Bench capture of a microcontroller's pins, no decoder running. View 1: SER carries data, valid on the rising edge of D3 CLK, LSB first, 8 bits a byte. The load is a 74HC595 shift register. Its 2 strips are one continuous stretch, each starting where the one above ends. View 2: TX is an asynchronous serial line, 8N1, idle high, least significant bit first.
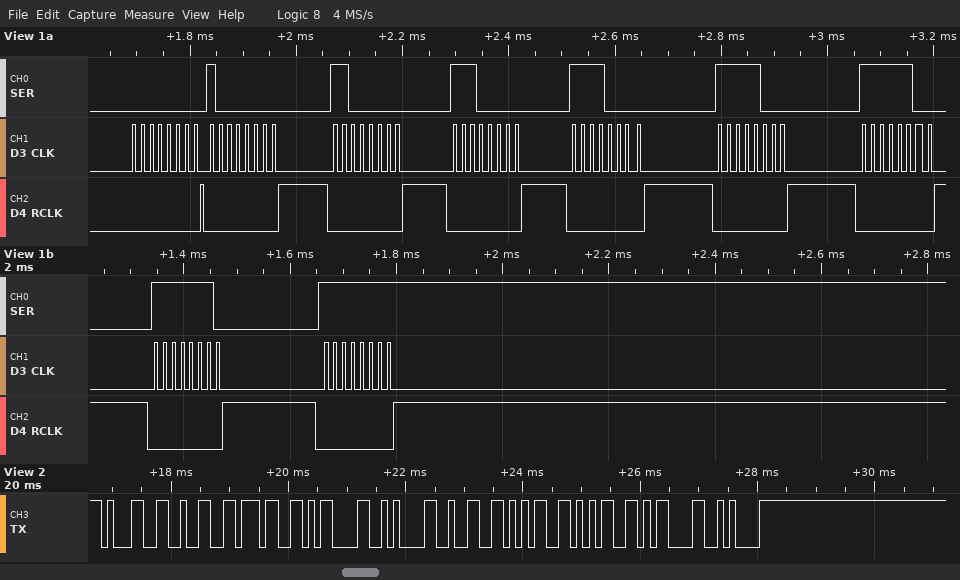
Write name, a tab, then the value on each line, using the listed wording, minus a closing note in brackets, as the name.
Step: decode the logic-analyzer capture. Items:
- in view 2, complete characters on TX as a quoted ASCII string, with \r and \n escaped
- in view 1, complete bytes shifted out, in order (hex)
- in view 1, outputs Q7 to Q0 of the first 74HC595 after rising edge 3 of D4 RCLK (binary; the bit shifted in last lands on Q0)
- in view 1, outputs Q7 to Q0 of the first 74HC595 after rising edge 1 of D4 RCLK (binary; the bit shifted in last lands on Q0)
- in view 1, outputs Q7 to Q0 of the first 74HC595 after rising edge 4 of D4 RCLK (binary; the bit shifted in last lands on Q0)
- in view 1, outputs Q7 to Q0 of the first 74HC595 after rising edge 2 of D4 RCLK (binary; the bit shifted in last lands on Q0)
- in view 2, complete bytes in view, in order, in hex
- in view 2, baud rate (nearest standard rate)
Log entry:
in view 2, complete characters on TX as a quoted ASCII string, with \r and \n escaped	"127\r\n255\r\n"
in view 1, complete bytes shifted out, in order	00 01 03 07 0F 1F 3F 7F FF
in view 1, outputs Q7 to Q0 of the first 74HC595 after rising edge 3 of D4 RCLK	11000000
in view 1, outputs Q7 to Q0 of the first 74HC595 after rising edge 1 of D4 RCLK	00000000
in view 1, outputs Q7 to Q0 of the first 74HC595 after rising edge 4 of D4 RCLK	11100000
in view 1, outputs Q7 to Q0 of the first 74HC595 after rising edge 2 of D4 RCLK	10000000
in view 2, complete bytes in view, in order, in hex	31 32 37 0D 0A 32 35 35 0D 0A
in view 2, baud rate	9600 baud
